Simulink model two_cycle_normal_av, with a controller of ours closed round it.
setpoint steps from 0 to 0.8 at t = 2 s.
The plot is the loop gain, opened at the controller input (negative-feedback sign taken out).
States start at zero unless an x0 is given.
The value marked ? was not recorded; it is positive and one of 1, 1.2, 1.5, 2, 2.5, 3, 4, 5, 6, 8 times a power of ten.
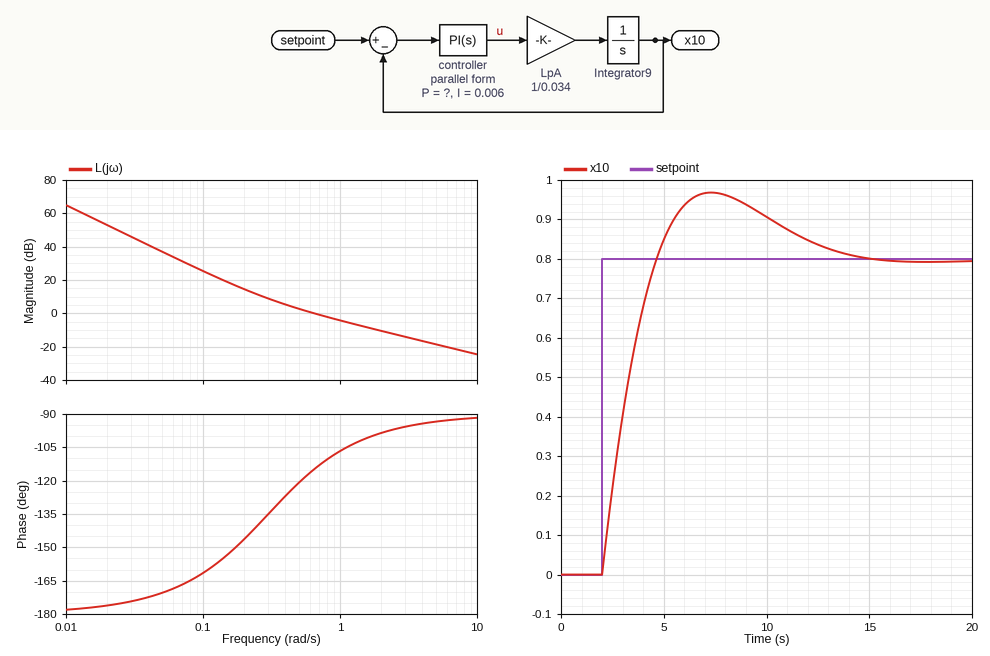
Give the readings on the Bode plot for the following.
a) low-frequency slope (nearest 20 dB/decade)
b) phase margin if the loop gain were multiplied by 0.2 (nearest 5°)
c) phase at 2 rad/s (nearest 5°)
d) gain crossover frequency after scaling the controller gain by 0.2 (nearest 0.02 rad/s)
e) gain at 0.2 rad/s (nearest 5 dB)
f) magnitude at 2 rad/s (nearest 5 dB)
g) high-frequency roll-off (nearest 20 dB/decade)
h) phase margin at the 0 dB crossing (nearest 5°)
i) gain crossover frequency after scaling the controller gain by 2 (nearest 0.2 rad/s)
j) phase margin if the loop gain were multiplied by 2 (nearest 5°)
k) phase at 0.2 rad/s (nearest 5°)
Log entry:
-40 dB/decade
35°
-100°
0.20 rad/s
15 dB
-10 dB
-20 dB/decade
65°
1.2 rad/s
75°
-145°
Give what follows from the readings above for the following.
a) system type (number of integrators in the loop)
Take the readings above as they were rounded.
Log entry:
2
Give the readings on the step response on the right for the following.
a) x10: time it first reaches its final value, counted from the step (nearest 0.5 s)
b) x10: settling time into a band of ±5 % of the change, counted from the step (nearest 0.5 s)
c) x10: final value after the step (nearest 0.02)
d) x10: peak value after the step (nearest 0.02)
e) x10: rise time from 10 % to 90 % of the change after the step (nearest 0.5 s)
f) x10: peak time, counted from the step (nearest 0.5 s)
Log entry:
2.5 s
10.5 s
0.80
0.96
2.0 s
5.5 s
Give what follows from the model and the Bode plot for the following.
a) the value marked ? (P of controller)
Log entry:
0.02
